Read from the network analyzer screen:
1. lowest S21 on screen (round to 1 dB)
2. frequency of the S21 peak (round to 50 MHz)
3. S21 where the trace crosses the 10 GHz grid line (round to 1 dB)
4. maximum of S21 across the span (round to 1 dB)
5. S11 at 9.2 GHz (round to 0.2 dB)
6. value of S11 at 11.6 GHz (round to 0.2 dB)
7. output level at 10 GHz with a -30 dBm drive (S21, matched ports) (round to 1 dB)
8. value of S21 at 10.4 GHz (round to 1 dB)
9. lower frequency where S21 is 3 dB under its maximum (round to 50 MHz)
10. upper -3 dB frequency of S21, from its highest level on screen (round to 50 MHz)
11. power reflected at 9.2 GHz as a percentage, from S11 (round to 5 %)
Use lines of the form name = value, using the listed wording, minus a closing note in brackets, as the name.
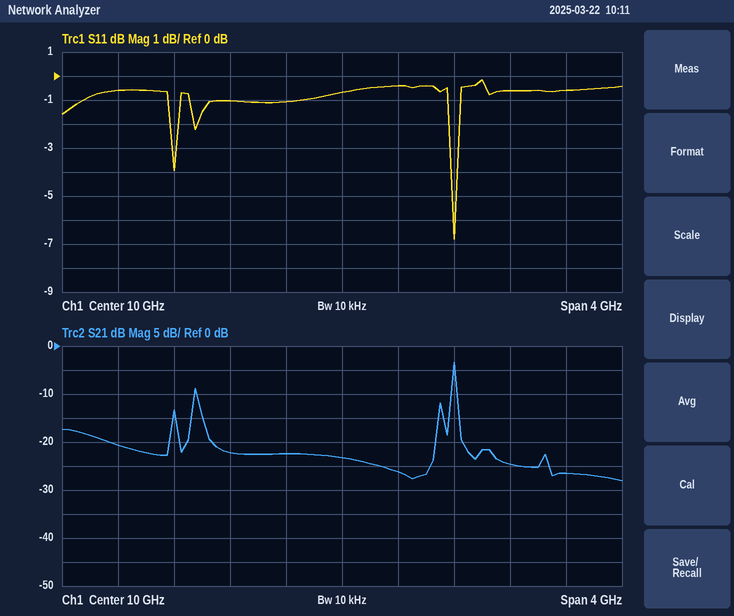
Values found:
lowest S21 on screen = -28 dB
frequency of the S21 peak = 10.80 GHz
S21 where the trace crosses the 10 GHz grid line = -23 dB
maximum of S21 across the span = -3 dB
S11 at 9.2 GHz = -1.0 dB
value of S11 at 11.6 GHz = -0.6 dB
output level at 10 GHz with a -30 dBm drive (S21, matched ports) = -53 dBm
value of S21 at 10.4 GHz = -26 dB
lower frequency where S21 is 3 dB under its maximum = 10.80 GHz
upper -3 dB frequency of S21, from its highest level on screen = 10.80 GHz
power reflected at 9.2 GHz as a percentage, from S11 = 80 %
